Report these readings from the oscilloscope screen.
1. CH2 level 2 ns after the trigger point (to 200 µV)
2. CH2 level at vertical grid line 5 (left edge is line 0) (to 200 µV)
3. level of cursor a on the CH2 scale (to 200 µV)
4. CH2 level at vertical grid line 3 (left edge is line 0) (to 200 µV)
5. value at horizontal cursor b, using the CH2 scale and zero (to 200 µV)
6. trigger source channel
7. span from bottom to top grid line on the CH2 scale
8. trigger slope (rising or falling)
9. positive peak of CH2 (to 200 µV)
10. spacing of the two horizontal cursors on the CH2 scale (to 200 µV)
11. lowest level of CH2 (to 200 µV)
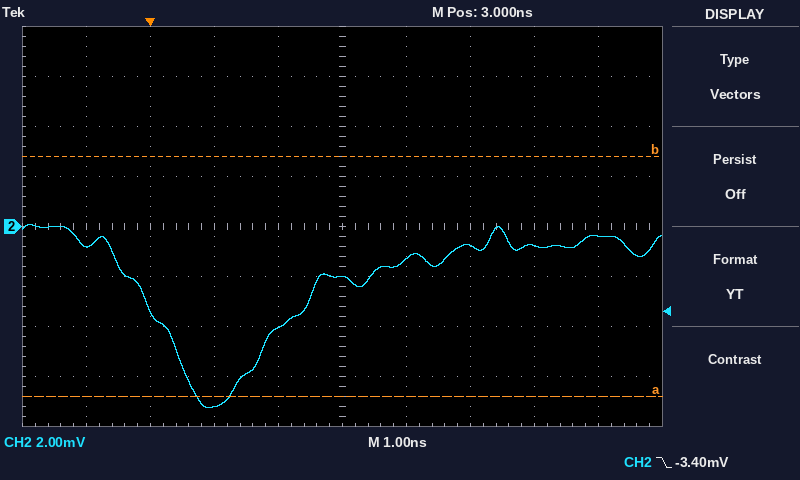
-4.0 mV
-2.0 mV
-6.8 mV
-7.2 mV
2.8 mV
CH2
16 mV
falling
0.0 mV
9.6 mV
-7.2 mV
